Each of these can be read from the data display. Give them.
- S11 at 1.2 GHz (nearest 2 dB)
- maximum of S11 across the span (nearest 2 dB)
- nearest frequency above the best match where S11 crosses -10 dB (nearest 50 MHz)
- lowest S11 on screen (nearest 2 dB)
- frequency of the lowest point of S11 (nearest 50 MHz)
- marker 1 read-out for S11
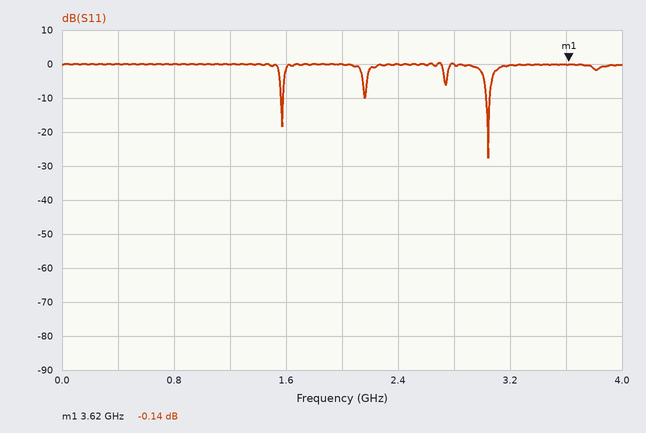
0 dB
0 dB
3.05 GHz
-28 dB
3.05 GHz
-0.14 dB
